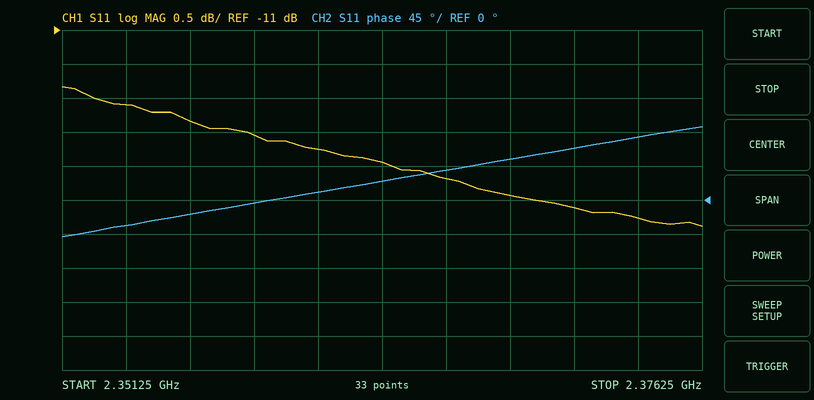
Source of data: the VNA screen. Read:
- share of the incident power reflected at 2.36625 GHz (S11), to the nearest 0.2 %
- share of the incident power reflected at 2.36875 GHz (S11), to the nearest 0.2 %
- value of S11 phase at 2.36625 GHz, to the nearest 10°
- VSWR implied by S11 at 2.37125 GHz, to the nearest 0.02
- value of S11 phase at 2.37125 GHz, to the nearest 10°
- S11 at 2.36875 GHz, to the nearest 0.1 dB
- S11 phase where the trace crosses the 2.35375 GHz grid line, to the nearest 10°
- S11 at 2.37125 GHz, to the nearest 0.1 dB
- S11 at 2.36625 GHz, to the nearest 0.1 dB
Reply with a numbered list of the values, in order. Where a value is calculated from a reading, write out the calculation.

1. 10^(-13.2/10) ≈ 4.8 %
2. 10^(-13.4/10) ≈ 4.6 %
3. 40°
4. |Γ| = 10^(-13.6/20) = 0.2089; VSWR = (1 + 0.2089)/(1 − 0.2089) ≈ 1.53, so 1.52 to the nearest 0.02
5. 70°
6. -13.4 dB
7. -30°
8. -13.6 dB
9. -13.2 dB
